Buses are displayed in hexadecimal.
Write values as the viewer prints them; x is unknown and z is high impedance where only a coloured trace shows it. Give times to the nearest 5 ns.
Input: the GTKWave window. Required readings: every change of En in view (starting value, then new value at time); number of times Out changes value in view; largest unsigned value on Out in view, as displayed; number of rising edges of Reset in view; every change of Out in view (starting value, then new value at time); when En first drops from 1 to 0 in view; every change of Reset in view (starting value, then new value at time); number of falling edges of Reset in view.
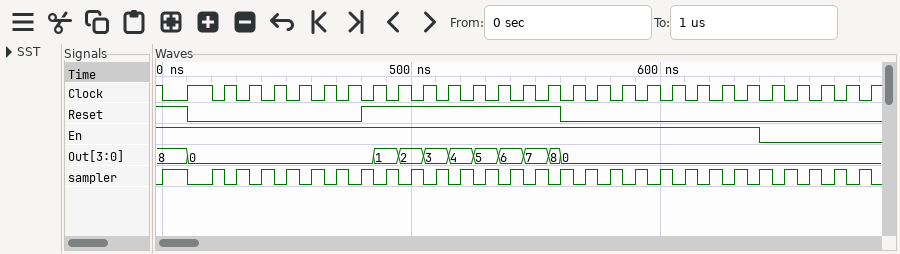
1, 0 at 640 ns
10
8
1
8, 0 at 410 ns, 1 at 485 ns, 2 at 495 ns, 3 at 505 ns, 4 at 515 ns, 5 at 525 ns, 6 at 535 ns, 7 at 545 ns, 8 at 555 ns, 0 at 560 ns
640 ns
1, 0 at 410 ns, 1 at 480 ns, 0 at 560 ns
2
